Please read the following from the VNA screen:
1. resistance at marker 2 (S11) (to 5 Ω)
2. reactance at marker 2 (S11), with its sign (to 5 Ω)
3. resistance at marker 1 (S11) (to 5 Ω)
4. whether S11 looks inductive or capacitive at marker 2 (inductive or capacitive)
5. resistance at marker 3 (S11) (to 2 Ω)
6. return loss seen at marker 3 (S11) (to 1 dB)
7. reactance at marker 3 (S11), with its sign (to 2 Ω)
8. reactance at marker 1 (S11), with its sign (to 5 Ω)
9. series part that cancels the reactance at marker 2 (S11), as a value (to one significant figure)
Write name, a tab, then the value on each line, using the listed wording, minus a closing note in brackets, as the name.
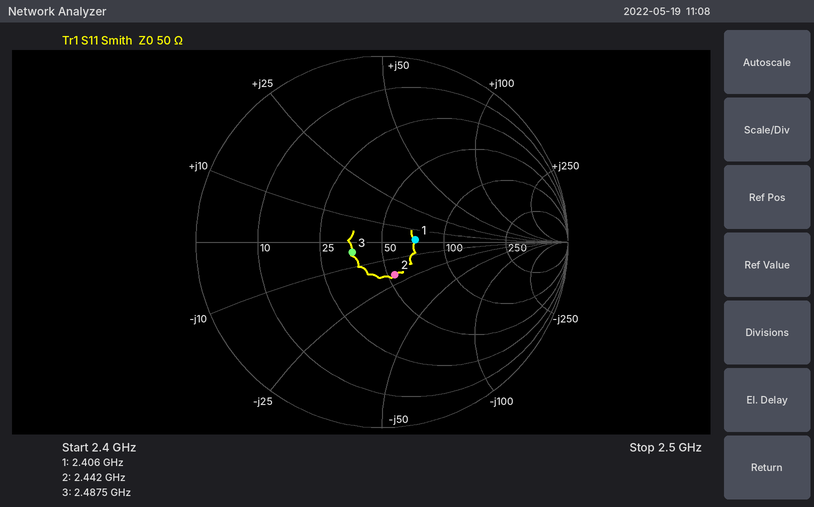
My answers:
resistance at marker 2 (S11)	55 Ω
reactance at marker 2 (S11), with its sign	-20 Ω
resistance at marker 1 (S11)	70 Ω
whether S11 looks inductive or capacitive at marker 2	capacitive
resistance at marker 3 (S11)	36 Ω
return loss seen at marker 3 (S11)	15 dB
reactance at marker 3 (S11), with its sign	-4 Ω
reactance at marker 1 (S11), with its sign	0 Ω
series part that cancels the reactance at marker 2 (S11), as a value	1 nH
